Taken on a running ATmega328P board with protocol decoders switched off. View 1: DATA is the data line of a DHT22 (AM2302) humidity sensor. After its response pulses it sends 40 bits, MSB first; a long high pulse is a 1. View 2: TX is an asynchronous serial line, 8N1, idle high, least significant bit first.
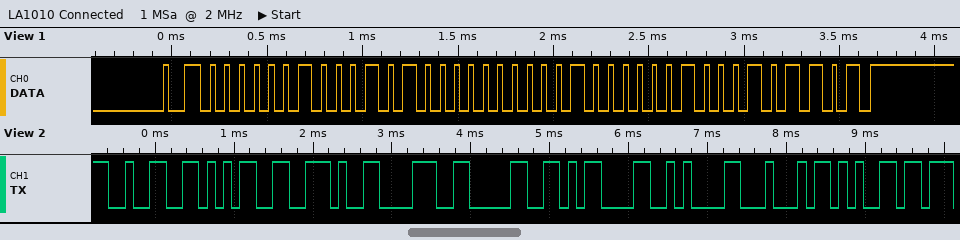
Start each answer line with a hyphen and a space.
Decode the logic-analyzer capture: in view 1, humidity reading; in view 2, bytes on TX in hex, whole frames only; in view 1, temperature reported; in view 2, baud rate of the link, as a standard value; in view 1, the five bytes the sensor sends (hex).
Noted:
- 55.2 %
- 32 35 2E 38 30 0D 0A 44 65
- 25.8 °C
- 9600 baud
- 02 28 01 02 2D
